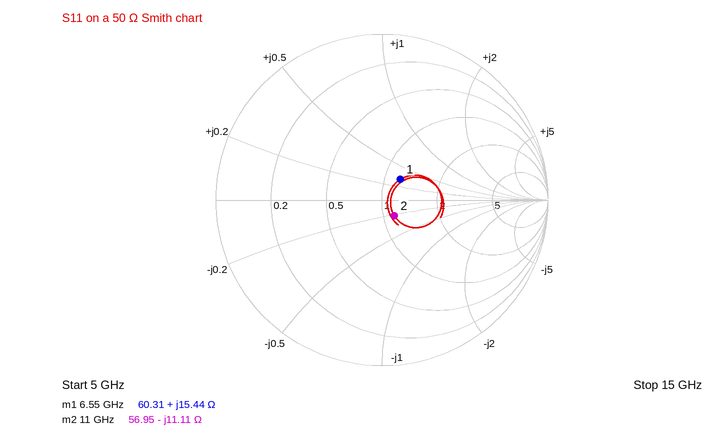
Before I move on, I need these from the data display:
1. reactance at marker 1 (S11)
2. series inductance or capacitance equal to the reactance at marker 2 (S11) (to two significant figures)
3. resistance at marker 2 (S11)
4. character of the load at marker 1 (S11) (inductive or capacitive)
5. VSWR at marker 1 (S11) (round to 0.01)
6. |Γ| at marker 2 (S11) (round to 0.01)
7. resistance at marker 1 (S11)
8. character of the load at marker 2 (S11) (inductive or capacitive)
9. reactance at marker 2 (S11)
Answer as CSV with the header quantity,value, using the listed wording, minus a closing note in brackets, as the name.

quantity,value
reactance at marker 1,+15.44 Ω
series inductance or capacitance equal to the reactance at marker 2 (S11),1.3 pF
resistance at marker 2,56.95 Ω
character of the load at marker 1 (S11),inductive
VSWR at marker 1 (S11),1.40
|Γ| at marker 2 (S11),0.12
resistance at marker 1,60.31 Ω
character of the load at marker 2 (S11),capacitive
reactance at marker 2,-11.11 Ω
